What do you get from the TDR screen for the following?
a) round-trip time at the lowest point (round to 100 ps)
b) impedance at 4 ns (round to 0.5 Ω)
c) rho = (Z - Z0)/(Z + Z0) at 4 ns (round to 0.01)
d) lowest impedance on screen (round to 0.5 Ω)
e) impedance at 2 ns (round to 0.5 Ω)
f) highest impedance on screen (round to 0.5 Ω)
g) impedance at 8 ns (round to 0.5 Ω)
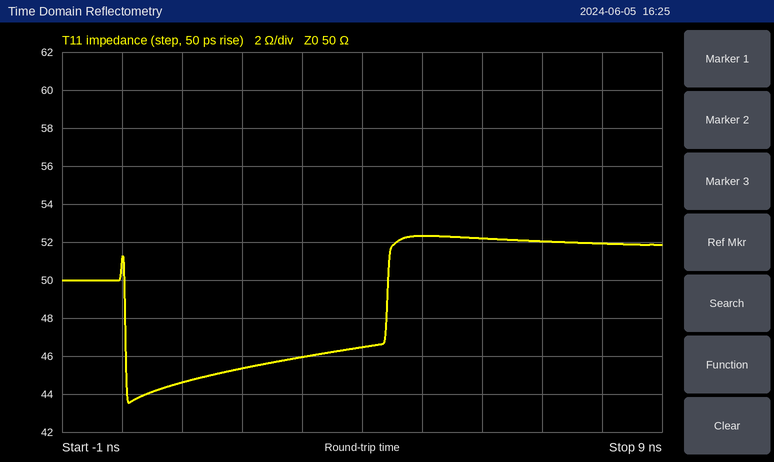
100 ps
46.5 Ω
-0.04
43.5 Ω
45.5 Ω
52.5 Ω
52.0 Ω
